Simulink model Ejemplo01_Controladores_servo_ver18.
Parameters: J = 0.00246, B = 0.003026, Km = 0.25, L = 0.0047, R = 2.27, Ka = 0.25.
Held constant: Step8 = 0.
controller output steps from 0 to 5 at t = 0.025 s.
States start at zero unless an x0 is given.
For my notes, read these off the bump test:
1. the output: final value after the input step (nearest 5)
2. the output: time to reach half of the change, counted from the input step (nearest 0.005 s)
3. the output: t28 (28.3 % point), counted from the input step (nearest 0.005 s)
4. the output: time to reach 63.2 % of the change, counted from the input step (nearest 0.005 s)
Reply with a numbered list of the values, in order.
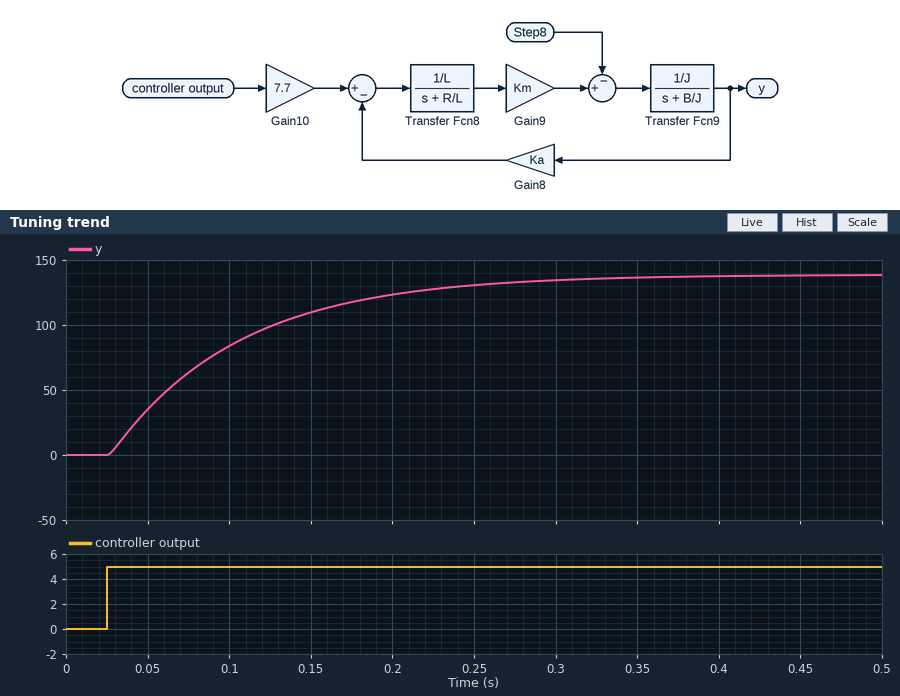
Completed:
1. 140
2. 0.055 s
3. 0.030 s
4. 0.080 s
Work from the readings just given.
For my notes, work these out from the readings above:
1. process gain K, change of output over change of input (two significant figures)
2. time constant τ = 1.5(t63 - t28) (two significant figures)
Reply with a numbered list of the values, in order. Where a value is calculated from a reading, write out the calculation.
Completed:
1. (140 - 0) / 5 = 28
2. 1.5 × (0.08 - 0.03) = 0.075 s
